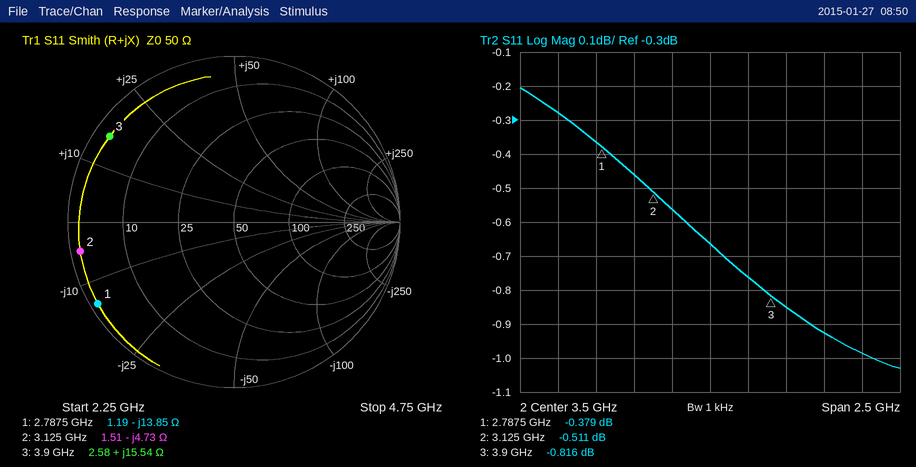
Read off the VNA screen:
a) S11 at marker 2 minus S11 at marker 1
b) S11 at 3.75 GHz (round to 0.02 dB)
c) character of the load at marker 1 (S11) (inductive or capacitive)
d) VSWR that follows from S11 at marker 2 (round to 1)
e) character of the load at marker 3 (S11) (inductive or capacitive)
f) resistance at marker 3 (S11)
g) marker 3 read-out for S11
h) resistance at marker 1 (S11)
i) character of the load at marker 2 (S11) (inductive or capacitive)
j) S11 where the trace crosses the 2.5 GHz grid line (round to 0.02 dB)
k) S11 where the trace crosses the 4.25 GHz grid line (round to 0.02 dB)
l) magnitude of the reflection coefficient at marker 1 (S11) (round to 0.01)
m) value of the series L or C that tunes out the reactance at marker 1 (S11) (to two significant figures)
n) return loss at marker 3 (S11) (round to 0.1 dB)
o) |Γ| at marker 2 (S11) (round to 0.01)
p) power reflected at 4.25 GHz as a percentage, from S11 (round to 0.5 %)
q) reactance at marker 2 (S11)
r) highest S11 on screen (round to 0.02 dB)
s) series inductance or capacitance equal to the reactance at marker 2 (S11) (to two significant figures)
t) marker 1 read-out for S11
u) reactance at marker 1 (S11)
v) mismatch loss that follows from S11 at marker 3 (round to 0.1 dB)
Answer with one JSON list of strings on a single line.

["-0.132 dB", "-0.76 dB", "capacitive", "34", "inductive", "2.58 Ω", "-0.816 dB", "1.19 Ω", "capacitive", "-0.28 dB", "-0.92 dB", "0.96", "790 pH", "0.8 dB", "0.94", "81.0 %", "-4.73 Ω", "-0.20 dB", "11 pF", "-0.379 dB", "-13.85 Ω", "7.7 dB"]
